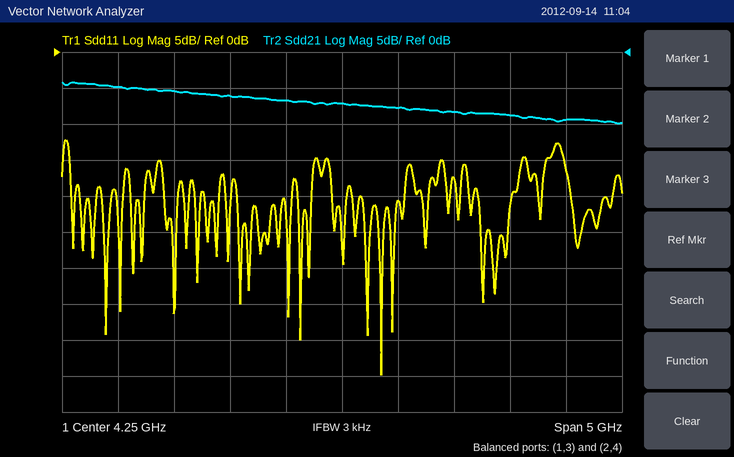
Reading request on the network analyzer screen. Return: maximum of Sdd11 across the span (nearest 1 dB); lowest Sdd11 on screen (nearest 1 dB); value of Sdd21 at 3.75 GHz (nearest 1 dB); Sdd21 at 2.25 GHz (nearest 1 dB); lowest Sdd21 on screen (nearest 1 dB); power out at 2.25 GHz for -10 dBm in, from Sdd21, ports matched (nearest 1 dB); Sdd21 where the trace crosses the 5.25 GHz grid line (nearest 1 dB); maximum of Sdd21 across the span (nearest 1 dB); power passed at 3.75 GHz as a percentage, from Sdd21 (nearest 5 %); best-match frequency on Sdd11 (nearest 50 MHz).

-12 dB
-45 dB
-7 dB
-5 dB
-10 dB
-15 dBm
-8 dB
-4 dB
20 %
4.60 GHz
